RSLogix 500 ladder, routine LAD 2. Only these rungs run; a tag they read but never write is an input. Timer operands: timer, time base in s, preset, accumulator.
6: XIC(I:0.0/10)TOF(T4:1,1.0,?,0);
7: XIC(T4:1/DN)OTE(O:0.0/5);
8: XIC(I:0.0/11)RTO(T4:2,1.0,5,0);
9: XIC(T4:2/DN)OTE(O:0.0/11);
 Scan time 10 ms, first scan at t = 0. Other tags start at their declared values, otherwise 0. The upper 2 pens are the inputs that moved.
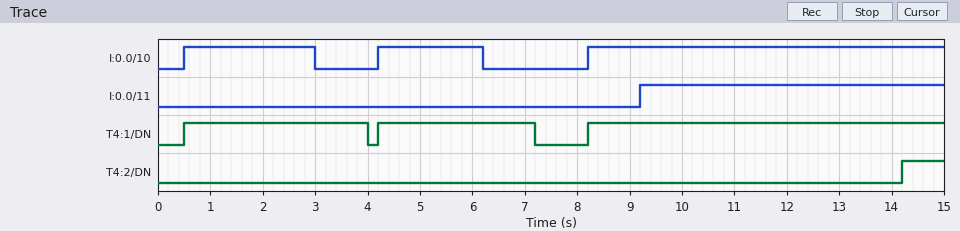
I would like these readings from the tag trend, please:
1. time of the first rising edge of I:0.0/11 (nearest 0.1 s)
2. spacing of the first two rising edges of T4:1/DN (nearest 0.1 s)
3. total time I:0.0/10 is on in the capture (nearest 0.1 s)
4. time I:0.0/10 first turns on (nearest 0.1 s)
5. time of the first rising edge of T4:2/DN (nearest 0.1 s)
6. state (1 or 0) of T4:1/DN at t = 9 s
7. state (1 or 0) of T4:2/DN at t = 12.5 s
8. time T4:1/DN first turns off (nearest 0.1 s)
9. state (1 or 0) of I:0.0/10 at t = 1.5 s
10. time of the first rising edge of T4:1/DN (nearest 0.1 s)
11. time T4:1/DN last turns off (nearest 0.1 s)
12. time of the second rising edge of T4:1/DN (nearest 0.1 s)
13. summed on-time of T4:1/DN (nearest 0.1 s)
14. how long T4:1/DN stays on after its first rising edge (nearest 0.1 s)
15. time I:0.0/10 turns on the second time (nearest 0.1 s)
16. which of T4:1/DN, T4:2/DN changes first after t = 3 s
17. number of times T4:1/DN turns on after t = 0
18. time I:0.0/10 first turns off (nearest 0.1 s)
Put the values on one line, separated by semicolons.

9.2 s; 3.7 s; 11.3 s; 0.5 s; 14.2 s; 1; 0; 4.0 s; 1; 0.5 s; 7.2 s; 4.2 s; 13.3 s; 3.5 s; 4.2 s; T4:1/DN; 3; 3.0 s
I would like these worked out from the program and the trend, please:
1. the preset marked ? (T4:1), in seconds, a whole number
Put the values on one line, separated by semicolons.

1 s
